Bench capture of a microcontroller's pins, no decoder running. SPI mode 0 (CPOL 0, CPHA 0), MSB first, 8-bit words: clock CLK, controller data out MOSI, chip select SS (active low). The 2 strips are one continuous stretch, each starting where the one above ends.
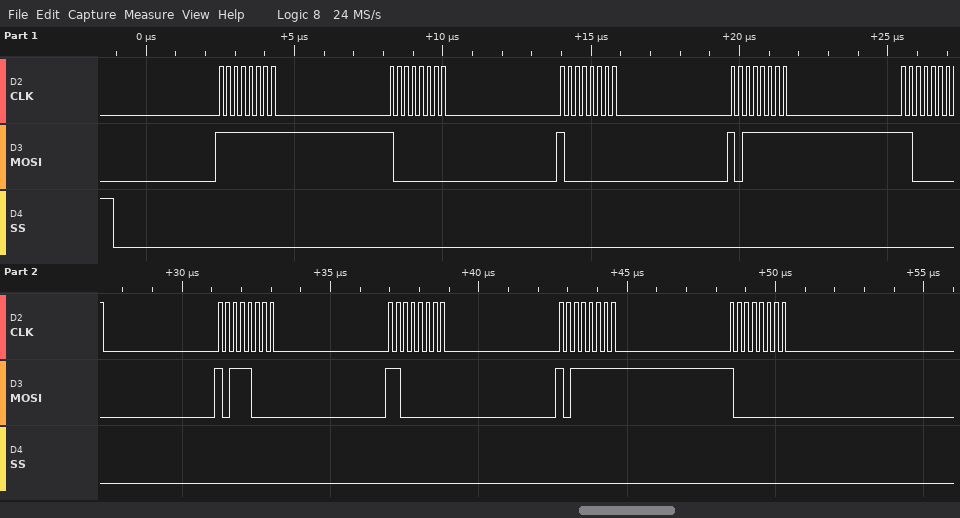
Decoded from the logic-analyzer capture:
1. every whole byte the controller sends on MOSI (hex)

FF 80 80 BF C0 B8 C0 BF 80
